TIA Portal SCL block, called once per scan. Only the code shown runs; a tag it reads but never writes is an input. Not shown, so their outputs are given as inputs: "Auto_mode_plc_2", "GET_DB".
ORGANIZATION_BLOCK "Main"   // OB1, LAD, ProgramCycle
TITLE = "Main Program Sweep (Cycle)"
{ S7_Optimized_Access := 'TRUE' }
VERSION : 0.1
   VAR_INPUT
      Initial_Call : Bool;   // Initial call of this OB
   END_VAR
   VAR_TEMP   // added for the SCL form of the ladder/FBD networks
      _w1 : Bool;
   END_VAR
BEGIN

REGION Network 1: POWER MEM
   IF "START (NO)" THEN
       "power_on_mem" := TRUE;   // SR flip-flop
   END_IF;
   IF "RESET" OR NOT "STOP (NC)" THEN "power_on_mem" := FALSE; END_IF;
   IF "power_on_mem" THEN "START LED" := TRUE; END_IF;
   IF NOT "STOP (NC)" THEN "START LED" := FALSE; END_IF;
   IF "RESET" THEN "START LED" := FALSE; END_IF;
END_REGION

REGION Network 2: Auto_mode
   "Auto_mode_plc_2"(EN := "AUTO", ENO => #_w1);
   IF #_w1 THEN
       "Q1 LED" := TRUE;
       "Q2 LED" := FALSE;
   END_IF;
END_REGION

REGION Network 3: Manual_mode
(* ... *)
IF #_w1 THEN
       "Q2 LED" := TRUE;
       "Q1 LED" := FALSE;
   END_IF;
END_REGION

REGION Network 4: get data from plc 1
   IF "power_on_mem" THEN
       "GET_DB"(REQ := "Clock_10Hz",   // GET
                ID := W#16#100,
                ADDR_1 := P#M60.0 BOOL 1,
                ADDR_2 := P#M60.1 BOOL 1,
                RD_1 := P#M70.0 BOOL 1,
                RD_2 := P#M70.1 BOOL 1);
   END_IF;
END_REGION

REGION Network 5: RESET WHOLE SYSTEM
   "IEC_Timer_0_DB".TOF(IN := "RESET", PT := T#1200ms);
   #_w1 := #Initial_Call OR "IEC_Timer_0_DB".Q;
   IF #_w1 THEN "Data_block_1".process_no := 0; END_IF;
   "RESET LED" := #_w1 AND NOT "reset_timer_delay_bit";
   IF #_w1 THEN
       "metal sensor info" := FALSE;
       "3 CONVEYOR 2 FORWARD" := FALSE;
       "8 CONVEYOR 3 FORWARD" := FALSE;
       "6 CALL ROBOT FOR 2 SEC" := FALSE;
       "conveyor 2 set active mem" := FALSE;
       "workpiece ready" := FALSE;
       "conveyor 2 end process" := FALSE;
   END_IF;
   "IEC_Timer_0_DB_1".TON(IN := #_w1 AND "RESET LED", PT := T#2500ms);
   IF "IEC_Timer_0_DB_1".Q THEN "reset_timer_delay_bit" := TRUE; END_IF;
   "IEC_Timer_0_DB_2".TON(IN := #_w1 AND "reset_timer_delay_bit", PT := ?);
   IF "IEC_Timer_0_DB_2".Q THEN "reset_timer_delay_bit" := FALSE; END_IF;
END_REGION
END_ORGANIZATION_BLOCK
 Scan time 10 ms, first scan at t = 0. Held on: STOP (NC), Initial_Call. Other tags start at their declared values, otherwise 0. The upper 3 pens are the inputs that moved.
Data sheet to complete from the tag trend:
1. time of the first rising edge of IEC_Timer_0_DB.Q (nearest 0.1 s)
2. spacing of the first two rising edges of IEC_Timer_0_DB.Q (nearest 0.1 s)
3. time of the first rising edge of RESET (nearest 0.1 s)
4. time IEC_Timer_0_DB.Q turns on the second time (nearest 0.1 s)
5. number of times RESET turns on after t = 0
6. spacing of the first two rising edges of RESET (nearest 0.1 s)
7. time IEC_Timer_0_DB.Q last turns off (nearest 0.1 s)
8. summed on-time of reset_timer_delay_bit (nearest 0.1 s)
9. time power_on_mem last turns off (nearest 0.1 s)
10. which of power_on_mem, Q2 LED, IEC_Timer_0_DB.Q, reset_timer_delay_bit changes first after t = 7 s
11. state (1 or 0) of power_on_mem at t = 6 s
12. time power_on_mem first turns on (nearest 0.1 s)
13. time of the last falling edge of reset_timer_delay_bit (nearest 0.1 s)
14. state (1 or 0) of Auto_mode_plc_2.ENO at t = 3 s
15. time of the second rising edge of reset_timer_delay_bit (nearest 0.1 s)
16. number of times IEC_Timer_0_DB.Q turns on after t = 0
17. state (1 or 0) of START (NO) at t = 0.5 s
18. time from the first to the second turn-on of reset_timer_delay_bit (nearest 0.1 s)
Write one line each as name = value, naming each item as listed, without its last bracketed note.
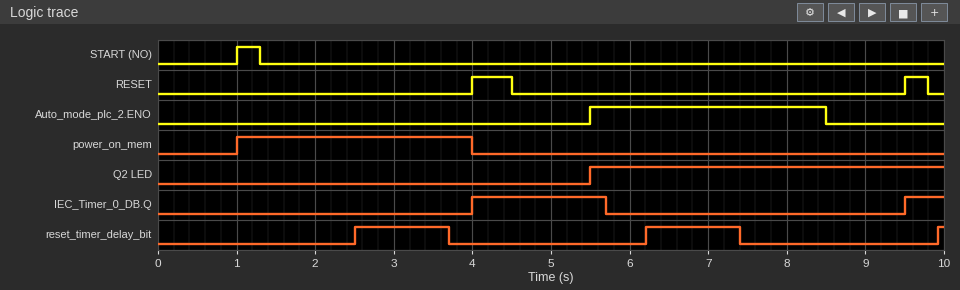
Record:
time of the first rising edge of IEC_Timer_0_DB.Q = 4.0 s
spacing of the first two rising edges of IEC_Timer_0_DB.Q = 5.5 s
time of the first rising edge of RESET = 4.0 s
time IEC_Timer_0_DB.Q turns on the second time = 9.5 s
number of times RESET turns on after t = 0 = 2
spacing of the first two rising edges of RESET = 5.5 s
time IEC_Timer_0_DB.Q last turns off = 5.7 s
summed on-time of reset_timer_delay_bit = 2.5 s
time power_on_mem last turns off = 4.0 s
which of power_on_mem, Q2 LED, IEC_Timer_0_DB.Q, reset_timer_delay_bit changes first after t = 7 s = reset_timer_delay_bit
state (1 or 0) of power_on_mem at t = 6 s = 0
time power_on_mem first turns on = 1.0 s
time of the last falling edge of reset_timer_delay_bit = 7.4 s
state (1 or 0) of Auto_mode_plc_2.ENO at t = 3 s = 0
time of the second rising edge of reset_timer_delay_bit = 6.2 s
number of times IEC_Timer_0_DB.Q turns on after t = 0 = 2
state (1 or 0) of START (NO) at t = 0.5 s = 0
time from the first to the second turn-on of reset_timer_delay_bit = 3.7 s
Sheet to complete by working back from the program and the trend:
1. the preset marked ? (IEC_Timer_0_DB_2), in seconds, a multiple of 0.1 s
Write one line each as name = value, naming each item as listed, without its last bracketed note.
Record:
the preset marked ? (IEC_Timer_0_DB_2), in seconds, a multiple of 0.1 s = 1.2 s
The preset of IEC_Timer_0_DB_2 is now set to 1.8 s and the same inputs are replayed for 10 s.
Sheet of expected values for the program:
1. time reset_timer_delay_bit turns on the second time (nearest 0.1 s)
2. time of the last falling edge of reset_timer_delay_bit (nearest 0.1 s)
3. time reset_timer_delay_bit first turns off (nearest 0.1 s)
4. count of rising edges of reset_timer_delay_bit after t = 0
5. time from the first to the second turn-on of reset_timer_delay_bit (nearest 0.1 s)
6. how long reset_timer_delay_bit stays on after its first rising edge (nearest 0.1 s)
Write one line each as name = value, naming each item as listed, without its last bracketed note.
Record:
time reset_timer_delay_bit turns on the second time = 6.8 s
time of the last falling edge of reset_timer_delay_bit = 8.6 s
time reset_timer_delay_bit first turns off = 4.3 s
count of rising edges of reset_timer_delay_bit after t = 0 = 2
time from the first to the second turn-on of reset_timer_delay_bit = 4.3 s
how long reset_timer_delay_bit stays on after its first rising edge = 1.8 s
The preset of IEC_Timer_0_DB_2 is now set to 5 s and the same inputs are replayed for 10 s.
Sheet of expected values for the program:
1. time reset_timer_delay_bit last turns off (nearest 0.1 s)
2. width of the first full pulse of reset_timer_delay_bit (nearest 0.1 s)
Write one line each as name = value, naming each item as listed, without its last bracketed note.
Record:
time reset_timer_delay_bit last turns off = 7.5 s
width of the first full pulse of reset_timer_delay_bit = 5.0 s
